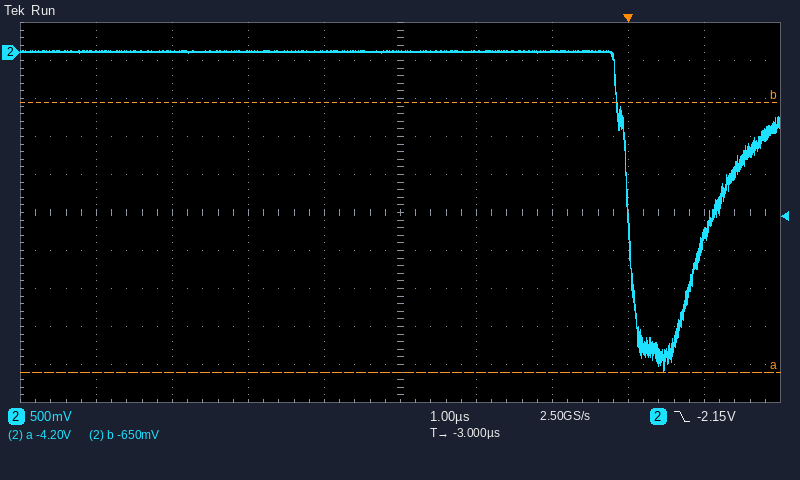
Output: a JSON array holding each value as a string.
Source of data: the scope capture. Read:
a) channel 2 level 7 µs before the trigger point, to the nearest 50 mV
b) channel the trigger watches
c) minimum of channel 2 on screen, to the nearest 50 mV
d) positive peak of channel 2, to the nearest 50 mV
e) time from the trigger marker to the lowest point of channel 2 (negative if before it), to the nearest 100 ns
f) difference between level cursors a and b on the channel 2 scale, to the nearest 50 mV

["0 mV", "channel 2", "-4.20 V", "50 mV", "+500 ns", "3.55 V"]
